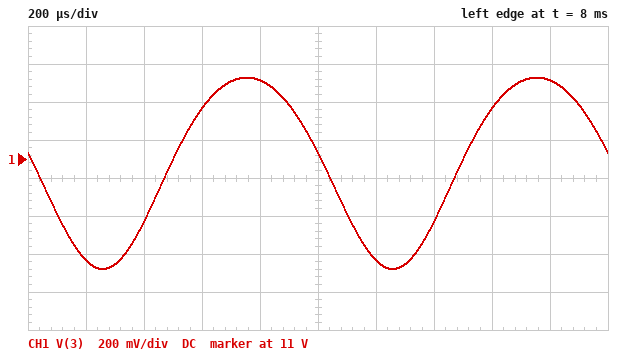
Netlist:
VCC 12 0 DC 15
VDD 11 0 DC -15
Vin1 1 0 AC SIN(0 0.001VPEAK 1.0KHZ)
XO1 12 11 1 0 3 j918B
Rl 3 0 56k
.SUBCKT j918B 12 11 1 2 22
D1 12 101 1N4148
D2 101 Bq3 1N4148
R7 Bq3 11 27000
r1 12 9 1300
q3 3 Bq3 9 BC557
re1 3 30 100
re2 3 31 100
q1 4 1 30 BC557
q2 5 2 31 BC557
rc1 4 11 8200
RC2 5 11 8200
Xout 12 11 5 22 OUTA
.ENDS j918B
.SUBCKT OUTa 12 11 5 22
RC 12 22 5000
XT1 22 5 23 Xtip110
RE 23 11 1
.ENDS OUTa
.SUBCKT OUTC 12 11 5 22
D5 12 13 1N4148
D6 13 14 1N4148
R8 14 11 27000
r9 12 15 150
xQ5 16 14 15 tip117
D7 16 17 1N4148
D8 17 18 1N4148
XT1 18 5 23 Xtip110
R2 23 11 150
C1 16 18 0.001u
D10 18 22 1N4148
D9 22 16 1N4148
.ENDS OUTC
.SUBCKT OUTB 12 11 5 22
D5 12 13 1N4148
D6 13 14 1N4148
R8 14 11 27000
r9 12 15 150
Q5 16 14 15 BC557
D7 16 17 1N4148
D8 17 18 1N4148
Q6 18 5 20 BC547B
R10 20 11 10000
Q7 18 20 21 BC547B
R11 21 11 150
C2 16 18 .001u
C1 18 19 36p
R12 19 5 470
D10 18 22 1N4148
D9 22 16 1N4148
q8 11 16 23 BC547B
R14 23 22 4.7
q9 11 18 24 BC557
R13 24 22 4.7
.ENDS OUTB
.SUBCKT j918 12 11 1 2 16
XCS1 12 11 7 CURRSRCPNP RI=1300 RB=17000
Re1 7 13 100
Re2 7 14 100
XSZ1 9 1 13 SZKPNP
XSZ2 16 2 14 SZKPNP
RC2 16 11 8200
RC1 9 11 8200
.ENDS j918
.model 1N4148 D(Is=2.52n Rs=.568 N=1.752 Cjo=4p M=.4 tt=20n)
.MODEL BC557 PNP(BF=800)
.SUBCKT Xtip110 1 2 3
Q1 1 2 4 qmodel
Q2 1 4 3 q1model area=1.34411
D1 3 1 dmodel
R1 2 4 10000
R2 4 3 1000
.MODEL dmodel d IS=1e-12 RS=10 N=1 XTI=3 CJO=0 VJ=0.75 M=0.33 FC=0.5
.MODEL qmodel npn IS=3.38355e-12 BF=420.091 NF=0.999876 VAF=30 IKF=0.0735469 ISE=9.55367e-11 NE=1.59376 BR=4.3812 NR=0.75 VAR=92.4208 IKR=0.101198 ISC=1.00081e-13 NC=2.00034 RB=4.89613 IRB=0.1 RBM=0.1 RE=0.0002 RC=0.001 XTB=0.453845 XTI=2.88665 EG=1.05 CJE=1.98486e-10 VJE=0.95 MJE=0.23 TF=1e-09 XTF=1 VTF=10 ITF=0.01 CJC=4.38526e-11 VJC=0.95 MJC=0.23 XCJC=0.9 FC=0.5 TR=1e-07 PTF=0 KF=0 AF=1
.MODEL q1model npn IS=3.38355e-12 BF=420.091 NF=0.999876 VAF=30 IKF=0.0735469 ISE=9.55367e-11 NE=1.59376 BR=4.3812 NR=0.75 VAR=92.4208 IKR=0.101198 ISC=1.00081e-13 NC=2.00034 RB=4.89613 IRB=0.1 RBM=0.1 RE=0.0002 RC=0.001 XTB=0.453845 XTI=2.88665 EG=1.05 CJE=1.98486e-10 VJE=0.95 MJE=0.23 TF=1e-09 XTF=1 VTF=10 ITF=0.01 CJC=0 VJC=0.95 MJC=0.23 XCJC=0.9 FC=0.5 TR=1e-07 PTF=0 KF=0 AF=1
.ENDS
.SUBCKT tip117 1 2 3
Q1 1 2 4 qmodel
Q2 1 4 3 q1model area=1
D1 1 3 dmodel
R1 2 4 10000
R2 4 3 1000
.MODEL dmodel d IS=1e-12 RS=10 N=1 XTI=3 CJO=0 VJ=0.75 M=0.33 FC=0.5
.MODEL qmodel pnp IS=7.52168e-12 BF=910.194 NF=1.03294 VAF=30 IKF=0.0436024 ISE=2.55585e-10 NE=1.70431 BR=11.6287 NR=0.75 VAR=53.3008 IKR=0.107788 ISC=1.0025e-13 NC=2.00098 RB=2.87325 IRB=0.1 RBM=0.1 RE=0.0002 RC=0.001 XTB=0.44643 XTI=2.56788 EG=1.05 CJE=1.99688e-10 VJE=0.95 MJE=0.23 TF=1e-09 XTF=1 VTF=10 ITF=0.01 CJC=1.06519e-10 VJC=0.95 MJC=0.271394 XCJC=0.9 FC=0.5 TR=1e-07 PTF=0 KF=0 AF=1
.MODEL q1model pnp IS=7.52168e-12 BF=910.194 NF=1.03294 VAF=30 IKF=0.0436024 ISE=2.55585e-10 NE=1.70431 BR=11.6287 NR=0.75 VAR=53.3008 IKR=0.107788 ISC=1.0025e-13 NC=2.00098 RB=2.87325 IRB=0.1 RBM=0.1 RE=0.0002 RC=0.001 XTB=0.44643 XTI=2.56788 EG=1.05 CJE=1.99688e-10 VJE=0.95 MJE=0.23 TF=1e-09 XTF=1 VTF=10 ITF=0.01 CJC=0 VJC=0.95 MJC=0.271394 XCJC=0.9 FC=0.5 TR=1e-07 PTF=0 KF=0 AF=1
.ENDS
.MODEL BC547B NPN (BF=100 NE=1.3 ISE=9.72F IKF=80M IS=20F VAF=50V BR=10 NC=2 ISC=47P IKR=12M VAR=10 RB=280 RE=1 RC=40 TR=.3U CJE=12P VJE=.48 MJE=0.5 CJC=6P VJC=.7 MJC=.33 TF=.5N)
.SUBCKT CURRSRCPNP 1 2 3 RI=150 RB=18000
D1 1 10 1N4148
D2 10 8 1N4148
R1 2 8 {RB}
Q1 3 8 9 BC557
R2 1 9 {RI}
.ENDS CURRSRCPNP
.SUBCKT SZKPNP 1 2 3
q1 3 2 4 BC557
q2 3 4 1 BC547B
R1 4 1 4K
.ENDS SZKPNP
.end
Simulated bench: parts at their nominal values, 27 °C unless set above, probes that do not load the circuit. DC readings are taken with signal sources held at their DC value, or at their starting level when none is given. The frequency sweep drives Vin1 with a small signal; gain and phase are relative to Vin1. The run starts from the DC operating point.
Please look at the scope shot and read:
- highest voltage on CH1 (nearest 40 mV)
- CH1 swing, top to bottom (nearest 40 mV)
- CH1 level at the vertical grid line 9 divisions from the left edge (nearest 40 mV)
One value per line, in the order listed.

11.44 V
1.00 V
11.40 V
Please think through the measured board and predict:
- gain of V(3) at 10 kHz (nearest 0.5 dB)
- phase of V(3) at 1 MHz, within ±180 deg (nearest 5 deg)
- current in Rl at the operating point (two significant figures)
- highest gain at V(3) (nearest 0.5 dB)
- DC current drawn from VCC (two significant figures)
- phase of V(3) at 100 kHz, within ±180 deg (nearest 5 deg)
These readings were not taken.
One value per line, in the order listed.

53.5 dB
90 deg
200 µA
54.0 dB
2.2 mA
105 deg
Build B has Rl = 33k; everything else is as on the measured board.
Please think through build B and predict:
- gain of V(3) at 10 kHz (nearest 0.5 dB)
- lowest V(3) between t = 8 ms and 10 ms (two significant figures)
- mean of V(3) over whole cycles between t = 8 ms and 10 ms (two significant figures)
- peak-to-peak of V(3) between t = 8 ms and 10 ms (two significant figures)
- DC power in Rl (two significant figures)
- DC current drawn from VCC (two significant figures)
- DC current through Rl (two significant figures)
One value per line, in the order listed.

52.5 dB
9.9 V
10 V
930 mV
3.3 mW
2.3 mA
320 µA
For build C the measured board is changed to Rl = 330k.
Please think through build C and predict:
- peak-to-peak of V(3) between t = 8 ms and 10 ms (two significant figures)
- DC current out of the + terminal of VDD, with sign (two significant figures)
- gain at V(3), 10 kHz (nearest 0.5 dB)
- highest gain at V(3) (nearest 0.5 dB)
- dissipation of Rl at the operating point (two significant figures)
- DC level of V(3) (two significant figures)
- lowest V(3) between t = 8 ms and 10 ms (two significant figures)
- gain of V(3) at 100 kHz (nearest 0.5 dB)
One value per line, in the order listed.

1.1 V
-2.0 mA
54.0 dB
55.0 dB
420 µW
12 V
11 V
43.0 dB
